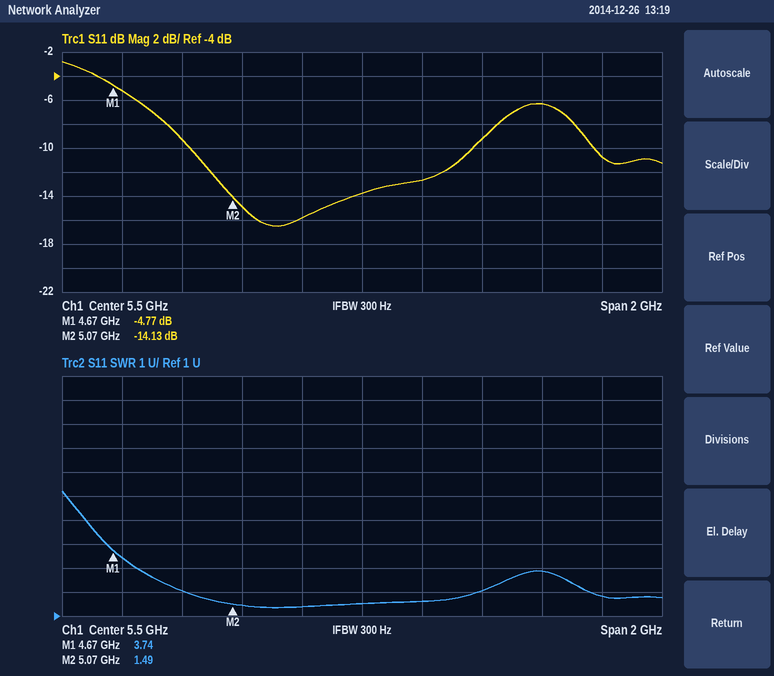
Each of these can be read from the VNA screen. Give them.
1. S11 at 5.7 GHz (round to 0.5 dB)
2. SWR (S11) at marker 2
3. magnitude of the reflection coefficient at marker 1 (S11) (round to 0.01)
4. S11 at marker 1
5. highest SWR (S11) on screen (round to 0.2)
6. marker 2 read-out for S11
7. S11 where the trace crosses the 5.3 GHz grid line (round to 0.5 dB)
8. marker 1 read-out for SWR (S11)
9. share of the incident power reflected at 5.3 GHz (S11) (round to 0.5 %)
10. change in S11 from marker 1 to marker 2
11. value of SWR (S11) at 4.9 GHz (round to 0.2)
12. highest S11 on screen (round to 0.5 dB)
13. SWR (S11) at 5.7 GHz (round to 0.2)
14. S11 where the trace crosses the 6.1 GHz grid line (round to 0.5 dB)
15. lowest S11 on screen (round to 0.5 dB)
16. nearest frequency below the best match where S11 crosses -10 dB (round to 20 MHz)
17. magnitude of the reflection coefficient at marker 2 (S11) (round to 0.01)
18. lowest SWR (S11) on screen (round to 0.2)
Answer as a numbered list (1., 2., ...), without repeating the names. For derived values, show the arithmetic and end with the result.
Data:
1. -12.5 dB
2. 1.49
3. 10^(-4.77/20) ≈ 0.58
4. -4.77 dB
5. 6.2
6. -14.13 dB
7. -16.0 dB
8. 3.74
9. 10^(-16/10) ≈ 2.5 %
10. -14.13 − (-4.77) = -9.36 dB
11. 2.0
12. -3.0 dB
13. 1.6
14. -6.5 dB
15. -16.5 dB
16. 4.92 GHz
17. 10^(-14.13/20) ≈ 0.20
18. 1.4
